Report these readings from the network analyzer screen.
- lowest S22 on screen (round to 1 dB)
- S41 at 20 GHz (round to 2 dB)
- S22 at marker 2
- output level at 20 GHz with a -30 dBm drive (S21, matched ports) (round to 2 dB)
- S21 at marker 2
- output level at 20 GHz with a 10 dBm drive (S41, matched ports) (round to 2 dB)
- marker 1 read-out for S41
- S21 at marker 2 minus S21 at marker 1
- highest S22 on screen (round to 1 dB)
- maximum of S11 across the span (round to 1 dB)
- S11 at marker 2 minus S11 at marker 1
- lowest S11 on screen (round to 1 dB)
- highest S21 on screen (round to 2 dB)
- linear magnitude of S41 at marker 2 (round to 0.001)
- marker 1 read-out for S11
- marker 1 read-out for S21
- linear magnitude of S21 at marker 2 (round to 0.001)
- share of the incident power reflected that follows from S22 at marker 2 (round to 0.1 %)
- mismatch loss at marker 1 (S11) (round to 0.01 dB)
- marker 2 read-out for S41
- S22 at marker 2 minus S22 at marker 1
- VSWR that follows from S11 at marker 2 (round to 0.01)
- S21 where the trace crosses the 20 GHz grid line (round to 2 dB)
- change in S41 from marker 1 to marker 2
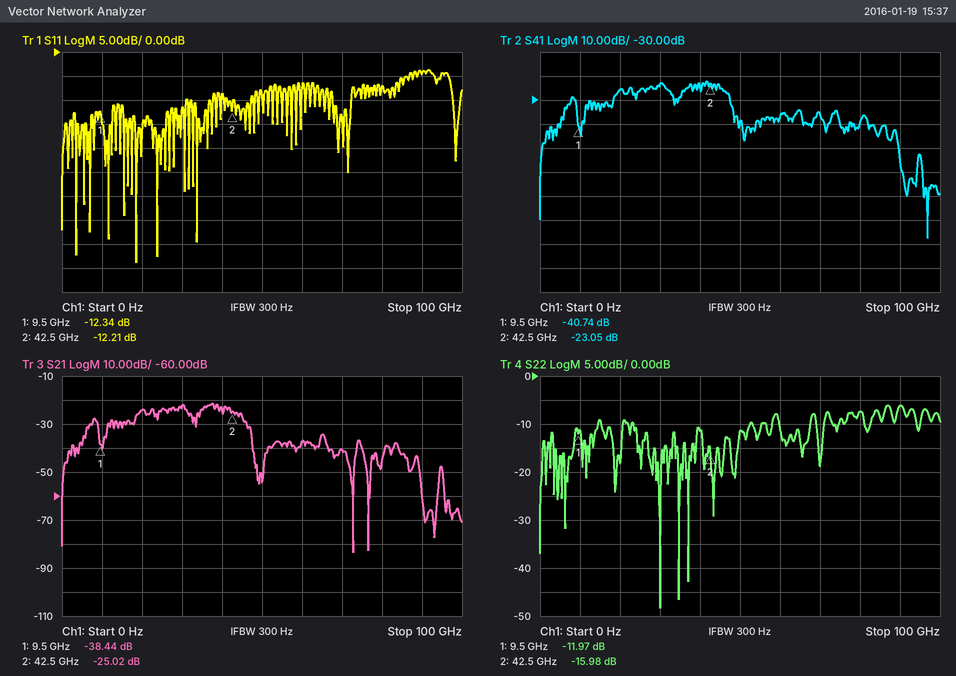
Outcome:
-48 dB
-26 dB
-15.98 dB
-54 dBm
-25.02 dB
-16 dBm
-40.74 dB
13.42 dB
-6 dB
-4 dB
0.13 dB
-44 dB
-22 dB
0.070
-12.34 dB
-38.44 dB
0.056
2.5 %
0.26 dB
-23.05 dB
-4.01 dB
1.65
-24 dB
17.69 dB
